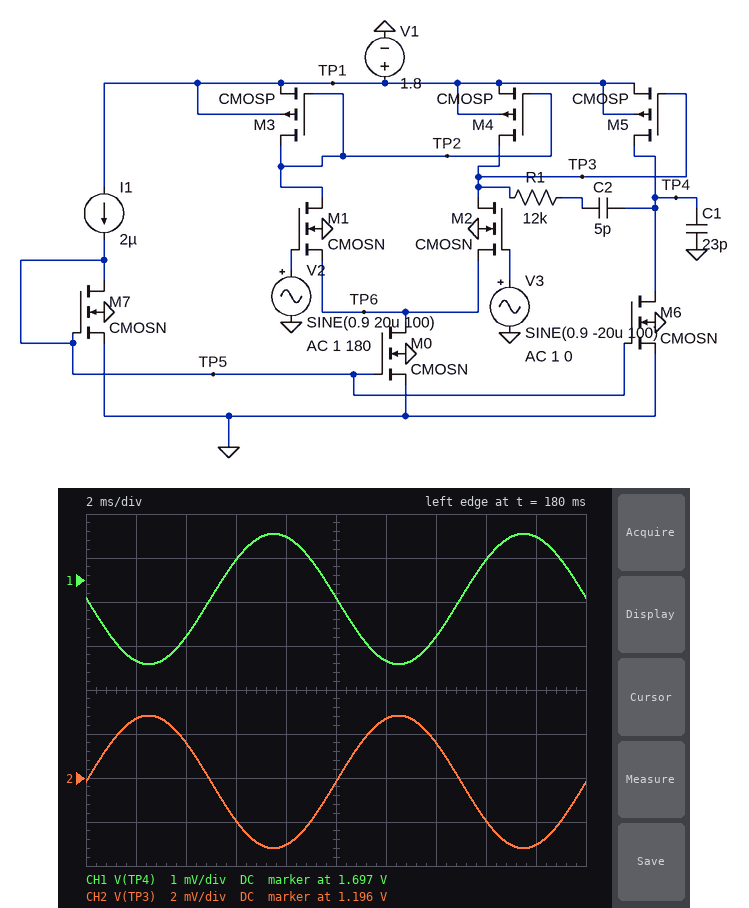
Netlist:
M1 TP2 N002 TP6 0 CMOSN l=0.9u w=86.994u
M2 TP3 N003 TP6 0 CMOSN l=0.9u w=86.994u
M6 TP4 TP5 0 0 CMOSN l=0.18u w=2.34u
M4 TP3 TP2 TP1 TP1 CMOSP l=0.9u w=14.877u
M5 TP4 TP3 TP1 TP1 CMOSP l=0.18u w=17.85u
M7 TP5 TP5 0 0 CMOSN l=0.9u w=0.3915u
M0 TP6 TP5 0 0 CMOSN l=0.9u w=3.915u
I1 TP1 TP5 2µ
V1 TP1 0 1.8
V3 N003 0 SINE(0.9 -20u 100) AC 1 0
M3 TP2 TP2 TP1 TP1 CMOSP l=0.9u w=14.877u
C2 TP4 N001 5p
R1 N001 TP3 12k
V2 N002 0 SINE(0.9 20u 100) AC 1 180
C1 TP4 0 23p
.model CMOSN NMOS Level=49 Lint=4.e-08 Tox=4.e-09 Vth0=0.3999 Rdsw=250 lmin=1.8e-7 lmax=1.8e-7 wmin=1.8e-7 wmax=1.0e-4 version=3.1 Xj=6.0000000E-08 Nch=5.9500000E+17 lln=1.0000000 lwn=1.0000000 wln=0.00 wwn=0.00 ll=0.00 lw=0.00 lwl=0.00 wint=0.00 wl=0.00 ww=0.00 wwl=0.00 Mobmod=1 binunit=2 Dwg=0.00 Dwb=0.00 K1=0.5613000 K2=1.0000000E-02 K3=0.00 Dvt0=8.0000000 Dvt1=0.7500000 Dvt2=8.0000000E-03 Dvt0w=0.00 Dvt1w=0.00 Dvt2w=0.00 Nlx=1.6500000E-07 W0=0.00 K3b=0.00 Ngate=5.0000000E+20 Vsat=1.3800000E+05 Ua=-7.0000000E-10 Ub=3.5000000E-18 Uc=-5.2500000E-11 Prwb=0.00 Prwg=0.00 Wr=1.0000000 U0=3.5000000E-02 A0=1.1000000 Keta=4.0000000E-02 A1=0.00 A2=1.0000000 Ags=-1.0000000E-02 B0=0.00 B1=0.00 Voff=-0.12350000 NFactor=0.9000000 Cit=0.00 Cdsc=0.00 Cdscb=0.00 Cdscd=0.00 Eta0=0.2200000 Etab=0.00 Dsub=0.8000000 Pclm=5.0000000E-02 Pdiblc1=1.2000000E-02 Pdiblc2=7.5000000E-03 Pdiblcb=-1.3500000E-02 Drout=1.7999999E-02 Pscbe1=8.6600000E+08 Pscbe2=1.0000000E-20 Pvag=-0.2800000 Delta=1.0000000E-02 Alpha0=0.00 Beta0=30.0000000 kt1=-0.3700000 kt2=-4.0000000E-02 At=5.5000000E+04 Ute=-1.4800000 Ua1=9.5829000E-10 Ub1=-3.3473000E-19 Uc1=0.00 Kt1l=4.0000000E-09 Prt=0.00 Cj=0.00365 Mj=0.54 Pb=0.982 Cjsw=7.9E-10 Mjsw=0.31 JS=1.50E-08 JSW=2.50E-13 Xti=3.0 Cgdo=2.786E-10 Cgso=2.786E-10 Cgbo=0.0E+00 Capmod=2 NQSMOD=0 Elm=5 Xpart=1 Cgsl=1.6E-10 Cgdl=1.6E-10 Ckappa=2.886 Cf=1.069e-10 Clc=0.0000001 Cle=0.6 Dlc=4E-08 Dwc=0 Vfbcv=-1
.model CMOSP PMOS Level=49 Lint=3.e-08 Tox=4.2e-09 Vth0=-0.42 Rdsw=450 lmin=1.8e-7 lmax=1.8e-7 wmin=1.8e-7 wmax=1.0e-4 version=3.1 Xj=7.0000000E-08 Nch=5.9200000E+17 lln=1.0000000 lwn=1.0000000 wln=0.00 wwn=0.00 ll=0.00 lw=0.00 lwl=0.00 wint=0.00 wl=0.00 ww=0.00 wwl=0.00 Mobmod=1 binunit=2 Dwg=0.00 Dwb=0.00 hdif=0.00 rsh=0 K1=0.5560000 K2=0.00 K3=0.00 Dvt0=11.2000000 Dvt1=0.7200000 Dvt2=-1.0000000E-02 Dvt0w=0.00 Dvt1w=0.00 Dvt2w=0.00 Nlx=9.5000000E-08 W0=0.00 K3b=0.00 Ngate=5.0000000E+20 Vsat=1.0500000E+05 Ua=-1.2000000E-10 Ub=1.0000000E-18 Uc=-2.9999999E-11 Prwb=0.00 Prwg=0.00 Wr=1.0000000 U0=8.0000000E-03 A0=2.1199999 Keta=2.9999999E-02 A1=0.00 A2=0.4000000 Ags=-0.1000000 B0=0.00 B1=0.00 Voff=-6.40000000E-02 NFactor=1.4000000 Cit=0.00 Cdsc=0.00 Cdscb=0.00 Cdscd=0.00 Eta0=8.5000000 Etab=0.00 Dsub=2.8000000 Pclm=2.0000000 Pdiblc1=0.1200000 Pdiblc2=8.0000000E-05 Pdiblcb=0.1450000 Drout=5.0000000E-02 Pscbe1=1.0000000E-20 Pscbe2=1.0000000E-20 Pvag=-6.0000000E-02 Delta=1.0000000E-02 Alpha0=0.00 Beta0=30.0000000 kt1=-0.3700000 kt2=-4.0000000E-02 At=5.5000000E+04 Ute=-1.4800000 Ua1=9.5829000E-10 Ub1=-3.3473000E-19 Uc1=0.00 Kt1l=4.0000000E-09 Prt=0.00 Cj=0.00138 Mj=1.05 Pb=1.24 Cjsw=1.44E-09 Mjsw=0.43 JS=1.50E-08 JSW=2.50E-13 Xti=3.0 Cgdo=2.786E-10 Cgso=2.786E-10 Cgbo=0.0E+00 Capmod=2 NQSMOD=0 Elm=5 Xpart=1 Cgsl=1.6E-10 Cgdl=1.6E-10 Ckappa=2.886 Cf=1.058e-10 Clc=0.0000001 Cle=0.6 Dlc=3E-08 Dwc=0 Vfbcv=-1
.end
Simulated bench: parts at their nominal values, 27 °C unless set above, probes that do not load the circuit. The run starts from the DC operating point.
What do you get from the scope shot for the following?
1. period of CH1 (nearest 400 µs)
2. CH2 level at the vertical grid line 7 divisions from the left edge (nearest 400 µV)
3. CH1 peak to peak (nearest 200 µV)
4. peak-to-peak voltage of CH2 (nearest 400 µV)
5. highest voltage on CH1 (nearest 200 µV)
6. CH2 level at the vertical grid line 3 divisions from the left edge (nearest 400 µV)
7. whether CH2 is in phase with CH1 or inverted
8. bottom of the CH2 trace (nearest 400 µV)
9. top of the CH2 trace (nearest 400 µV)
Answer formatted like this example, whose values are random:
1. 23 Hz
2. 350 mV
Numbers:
1. 10.0 ms
2. 1.1976 V
3. 3.0 mV
4. 6.0 mV
5. 1.6980 V
6. 1.1940 V
7. inverted
8. 1.1928 V
9. 1.1988 V
